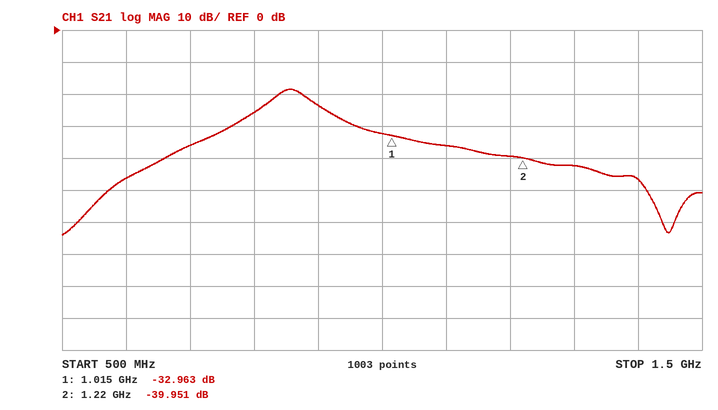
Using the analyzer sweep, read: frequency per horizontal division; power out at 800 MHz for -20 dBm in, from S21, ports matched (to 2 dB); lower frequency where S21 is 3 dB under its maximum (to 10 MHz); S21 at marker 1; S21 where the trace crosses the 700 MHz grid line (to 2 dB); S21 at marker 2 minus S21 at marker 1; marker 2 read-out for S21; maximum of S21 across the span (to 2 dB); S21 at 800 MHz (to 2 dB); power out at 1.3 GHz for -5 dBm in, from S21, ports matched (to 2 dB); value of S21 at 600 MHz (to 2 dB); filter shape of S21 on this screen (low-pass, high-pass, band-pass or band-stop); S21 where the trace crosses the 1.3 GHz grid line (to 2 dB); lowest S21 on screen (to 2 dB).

100 MHz
-46 dBm
830 MHz
-32.963 dB
-36 dB
-6.988 dB
-39.951 dB
-18 dB
-26 dB
-48 dBm
-46 dB
band-pass
-42 dB
-64 dB
